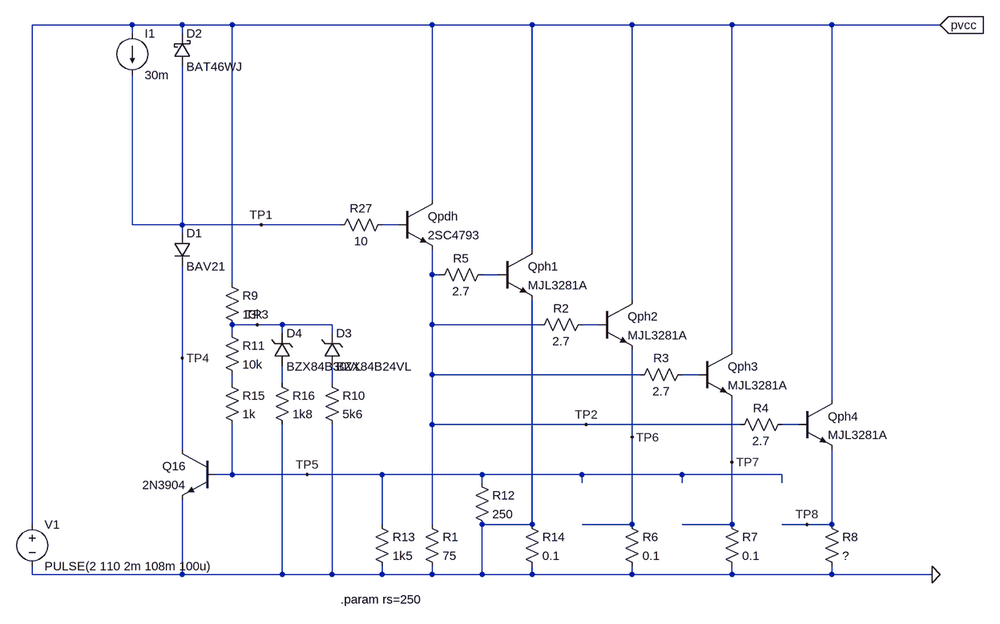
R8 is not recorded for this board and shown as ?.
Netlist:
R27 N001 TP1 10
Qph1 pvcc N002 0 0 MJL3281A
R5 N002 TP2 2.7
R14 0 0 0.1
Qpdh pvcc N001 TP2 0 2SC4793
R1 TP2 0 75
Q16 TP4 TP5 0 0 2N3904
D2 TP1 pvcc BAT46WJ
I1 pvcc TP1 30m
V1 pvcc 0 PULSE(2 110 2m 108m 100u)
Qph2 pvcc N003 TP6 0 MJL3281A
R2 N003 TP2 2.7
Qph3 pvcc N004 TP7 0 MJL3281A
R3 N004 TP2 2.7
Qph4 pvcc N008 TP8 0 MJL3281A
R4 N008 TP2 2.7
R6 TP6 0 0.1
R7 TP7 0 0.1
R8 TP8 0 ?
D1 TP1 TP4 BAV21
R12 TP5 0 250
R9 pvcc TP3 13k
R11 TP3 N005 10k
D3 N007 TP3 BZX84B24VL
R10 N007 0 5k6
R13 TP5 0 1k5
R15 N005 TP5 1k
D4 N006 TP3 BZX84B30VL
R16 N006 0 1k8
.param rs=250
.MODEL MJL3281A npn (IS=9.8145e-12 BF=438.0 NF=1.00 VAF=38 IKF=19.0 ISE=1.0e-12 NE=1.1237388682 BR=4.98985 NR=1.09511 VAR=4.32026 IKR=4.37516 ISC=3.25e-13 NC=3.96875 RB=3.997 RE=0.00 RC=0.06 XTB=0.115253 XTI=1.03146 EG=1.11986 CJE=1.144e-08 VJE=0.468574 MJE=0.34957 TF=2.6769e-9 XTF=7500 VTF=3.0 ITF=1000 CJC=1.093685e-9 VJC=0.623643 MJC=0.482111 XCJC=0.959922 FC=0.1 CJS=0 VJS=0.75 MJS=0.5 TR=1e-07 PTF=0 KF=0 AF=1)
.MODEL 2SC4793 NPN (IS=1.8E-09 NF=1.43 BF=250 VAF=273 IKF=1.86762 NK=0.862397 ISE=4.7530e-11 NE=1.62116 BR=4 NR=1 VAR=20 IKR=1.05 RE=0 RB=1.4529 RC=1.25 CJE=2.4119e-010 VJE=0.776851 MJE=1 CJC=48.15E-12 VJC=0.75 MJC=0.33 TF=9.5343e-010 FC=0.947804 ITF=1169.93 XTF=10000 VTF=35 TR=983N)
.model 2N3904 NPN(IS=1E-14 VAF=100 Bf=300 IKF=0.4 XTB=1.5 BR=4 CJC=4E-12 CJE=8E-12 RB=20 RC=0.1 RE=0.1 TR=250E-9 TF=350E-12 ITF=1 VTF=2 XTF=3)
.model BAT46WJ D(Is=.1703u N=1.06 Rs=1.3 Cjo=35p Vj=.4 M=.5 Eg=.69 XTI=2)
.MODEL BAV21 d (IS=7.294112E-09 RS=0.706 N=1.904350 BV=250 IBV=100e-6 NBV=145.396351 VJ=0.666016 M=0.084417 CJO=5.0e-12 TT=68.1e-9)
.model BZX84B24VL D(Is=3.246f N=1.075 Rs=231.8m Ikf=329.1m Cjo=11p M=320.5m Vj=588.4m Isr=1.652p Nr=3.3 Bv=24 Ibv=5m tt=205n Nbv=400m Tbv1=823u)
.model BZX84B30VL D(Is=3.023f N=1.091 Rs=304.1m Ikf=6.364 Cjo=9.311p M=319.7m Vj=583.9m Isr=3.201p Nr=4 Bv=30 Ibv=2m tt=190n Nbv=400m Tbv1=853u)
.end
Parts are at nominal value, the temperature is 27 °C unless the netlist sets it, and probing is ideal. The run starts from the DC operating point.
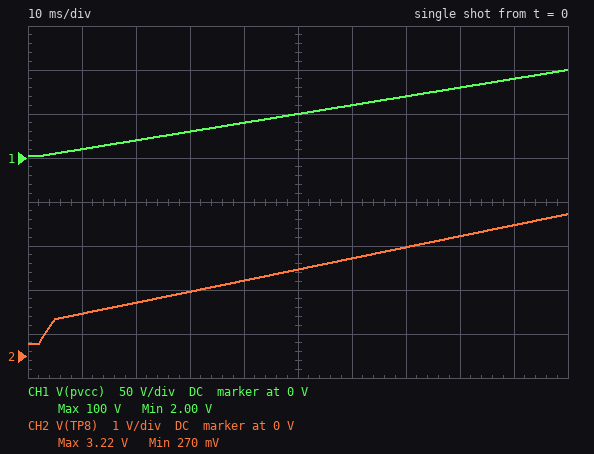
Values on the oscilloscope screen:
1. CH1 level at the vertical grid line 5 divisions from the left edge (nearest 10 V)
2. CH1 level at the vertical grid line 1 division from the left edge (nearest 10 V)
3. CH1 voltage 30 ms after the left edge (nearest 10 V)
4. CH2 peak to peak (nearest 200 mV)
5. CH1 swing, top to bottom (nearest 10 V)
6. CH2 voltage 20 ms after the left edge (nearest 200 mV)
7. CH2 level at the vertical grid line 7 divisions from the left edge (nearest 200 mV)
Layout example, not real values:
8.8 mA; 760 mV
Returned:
50 V; 10 V; 30 V; 3.0 V; 100 V; 1.2 V; 2.4 V
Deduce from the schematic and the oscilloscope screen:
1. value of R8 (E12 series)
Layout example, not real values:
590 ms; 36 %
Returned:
0.047 Ω
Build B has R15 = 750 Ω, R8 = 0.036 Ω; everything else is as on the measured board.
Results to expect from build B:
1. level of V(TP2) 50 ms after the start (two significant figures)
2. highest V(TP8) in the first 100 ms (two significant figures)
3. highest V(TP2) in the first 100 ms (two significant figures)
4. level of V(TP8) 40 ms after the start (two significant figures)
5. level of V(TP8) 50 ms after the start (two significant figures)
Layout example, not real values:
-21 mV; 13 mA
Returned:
4.5 V; 2.7 V; 5.7 V; 1.4 V; 1.6 V
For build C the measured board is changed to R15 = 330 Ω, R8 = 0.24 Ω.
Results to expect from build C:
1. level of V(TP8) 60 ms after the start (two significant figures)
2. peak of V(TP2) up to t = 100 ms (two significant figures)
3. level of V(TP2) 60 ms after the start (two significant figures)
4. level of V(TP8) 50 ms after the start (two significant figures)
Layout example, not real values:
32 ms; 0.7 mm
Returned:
4.3 V; 6.7 V; 5.6 V; 4.0 V
